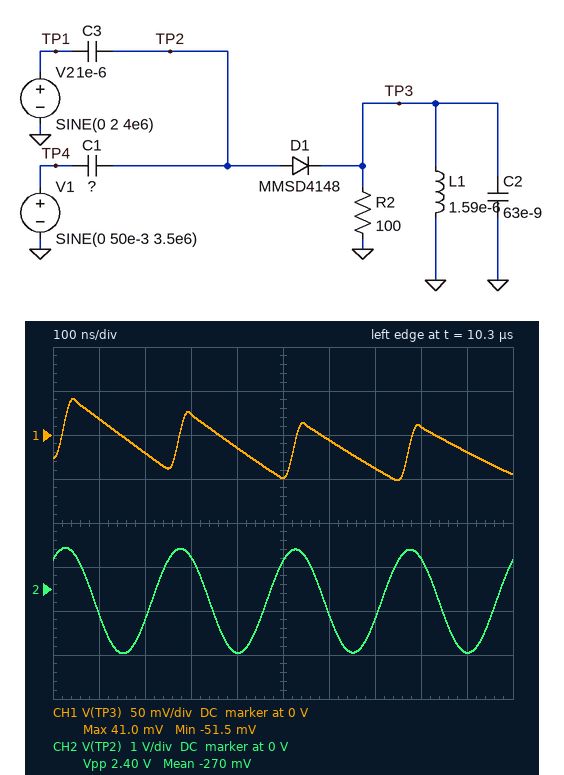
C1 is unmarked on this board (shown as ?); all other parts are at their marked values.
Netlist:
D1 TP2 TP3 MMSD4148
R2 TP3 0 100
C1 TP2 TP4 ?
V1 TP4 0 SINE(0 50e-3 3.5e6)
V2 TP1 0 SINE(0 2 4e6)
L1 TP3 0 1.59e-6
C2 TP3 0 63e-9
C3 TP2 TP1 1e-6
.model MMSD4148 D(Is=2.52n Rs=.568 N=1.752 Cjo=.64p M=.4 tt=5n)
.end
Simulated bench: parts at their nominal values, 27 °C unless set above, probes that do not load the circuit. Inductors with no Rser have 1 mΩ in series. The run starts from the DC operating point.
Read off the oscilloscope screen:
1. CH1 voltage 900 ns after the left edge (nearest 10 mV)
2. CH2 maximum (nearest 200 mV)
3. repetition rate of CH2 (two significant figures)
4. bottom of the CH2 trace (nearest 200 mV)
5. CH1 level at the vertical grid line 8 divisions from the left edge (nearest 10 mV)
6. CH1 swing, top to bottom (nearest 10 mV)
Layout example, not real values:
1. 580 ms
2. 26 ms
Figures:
1. -20 mV
2. 1.0 V
3. 4.0 MHz
4. -1.4 V
5. 10 mV
6. 90 mV
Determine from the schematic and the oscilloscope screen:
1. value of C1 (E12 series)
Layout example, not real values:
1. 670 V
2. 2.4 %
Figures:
1. 680 nF
